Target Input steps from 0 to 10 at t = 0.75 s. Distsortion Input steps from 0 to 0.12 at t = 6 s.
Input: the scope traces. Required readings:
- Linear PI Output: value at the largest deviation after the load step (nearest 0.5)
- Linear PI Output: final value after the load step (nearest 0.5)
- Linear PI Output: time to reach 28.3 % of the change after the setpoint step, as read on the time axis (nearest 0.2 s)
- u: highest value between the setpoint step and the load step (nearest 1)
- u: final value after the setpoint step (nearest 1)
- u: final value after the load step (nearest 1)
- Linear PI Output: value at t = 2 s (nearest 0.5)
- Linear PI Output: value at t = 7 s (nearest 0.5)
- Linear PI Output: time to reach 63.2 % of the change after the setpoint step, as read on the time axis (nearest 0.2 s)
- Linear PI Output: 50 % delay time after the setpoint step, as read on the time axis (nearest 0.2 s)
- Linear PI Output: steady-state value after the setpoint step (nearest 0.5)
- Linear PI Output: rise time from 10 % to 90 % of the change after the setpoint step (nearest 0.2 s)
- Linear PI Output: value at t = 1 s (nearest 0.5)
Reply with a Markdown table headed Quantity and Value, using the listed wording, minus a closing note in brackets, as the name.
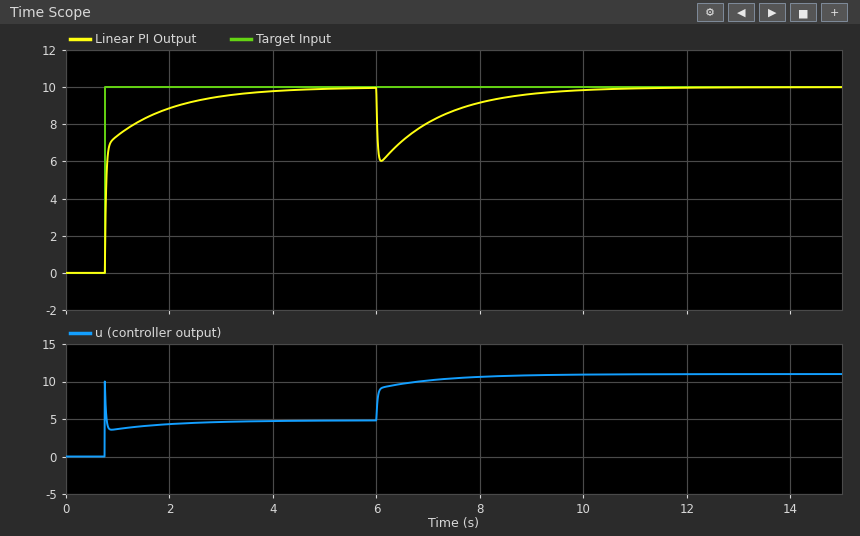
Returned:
| Quantity | Value |
|---|---|
| Linear PI Output: value at the largest deviation after the load step | 6.0 |
| Linear PI Output: final value after the load step | 10.0 |
| Linear PI Output: time to reach 28.3 % of the change after the setpoint step, as read on the time axis | 0.8 s |
| u: highest value between the setpoint step and the load step | 10 |
| u: final value after the setpoint step | 5 |
| u: final value after the load step | 11 |
| Linear PI Output: value at t = 2 s | 9.0 |
| Linear PI Output: value at t = 7 s | 8.0 |
| Linear PI Output: time to reach 63.2 % of the change after the setpoint step, as read on the time axis | 0.8 s |
| Linear PI Output: 50 % delay time after the setpoint step, as read on the time axis | 0.8 s |
| Linear PI Output: steady-state value after the setpoint step | 10.0 |
| Linear PI Output: rise time from 10 % to 90 % of the change after the setpoint step | 1.4 s |
| Linear PI Output: value at t = 1 s | 7.5 |
